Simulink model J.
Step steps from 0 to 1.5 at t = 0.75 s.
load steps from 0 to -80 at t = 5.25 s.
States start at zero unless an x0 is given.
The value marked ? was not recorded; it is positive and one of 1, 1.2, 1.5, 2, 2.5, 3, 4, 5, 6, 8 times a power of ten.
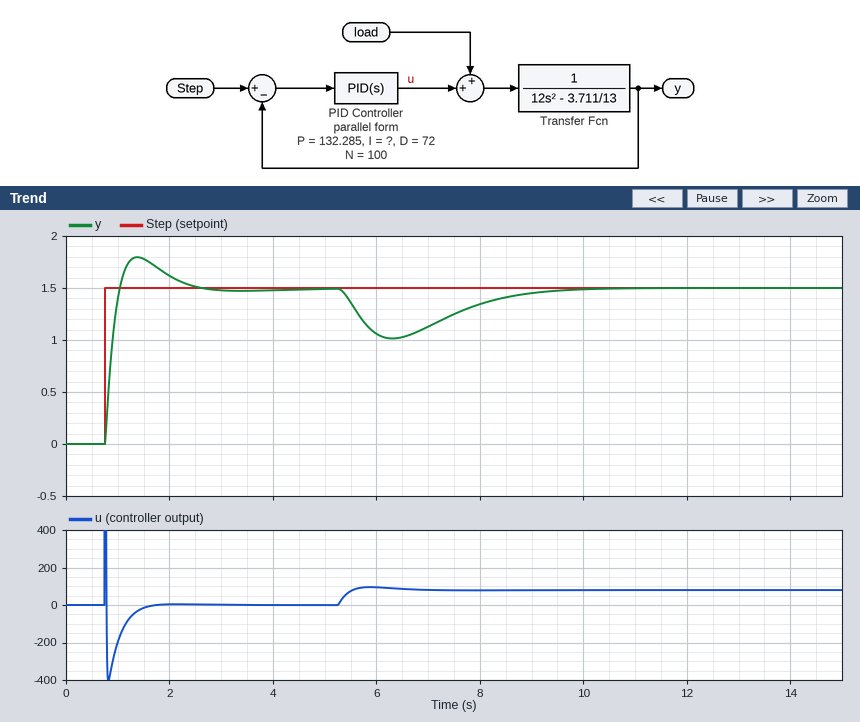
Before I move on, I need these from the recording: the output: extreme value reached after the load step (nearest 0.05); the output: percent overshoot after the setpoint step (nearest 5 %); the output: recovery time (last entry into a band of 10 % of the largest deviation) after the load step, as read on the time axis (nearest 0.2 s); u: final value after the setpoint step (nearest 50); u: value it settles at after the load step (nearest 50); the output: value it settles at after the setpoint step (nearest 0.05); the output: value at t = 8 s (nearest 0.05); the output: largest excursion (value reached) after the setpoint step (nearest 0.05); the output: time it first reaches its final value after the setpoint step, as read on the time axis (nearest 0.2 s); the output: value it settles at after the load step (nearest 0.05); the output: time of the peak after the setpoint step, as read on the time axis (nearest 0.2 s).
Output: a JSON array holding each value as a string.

["1.00", "20 %", "9.0 s", "0", "100", "1.50", "1.35", "1.80", "1.0 s", "1.50", "1.4 s"]
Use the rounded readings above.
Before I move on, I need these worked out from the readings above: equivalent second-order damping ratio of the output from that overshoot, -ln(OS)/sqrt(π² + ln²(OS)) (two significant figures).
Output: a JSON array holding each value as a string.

["0.46"]
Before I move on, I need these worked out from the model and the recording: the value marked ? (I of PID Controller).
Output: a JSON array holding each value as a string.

["80"]
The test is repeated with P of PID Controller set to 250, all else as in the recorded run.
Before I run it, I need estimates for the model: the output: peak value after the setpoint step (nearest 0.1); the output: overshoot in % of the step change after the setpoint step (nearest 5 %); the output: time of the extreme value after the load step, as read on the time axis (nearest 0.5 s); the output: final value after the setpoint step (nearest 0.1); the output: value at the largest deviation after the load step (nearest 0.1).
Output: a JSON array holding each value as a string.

["1.9", "25 %", "6.0 s", "1.5", "1.2"]
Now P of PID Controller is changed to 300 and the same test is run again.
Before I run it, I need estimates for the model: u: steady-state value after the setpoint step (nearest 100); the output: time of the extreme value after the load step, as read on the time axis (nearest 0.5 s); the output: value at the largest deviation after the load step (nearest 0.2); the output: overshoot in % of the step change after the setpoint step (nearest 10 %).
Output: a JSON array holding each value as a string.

["0", "6.0 s", "1.2", "30 %"]
